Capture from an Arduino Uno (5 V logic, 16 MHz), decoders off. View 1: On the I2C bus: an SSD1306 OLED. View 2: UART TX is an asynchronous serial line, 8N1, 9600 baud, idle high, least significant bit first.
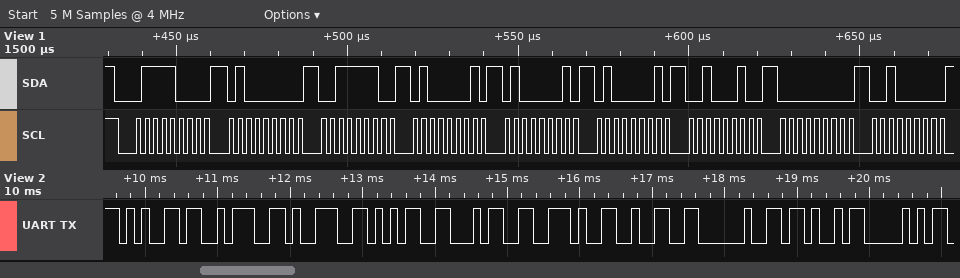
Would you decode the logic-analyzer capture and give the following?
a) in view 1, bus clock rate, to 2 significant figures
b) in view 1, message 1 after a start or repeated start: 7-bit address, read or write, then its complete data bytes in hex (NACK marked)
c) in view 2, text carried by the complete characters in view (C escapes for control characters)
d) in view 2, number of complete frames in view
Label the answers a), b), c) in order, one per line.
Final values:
a) 400 kHz
b) 0x3C write: 40 3E 41 41 41 22 00 20
c) "e:954.2 KP"
d) 10
